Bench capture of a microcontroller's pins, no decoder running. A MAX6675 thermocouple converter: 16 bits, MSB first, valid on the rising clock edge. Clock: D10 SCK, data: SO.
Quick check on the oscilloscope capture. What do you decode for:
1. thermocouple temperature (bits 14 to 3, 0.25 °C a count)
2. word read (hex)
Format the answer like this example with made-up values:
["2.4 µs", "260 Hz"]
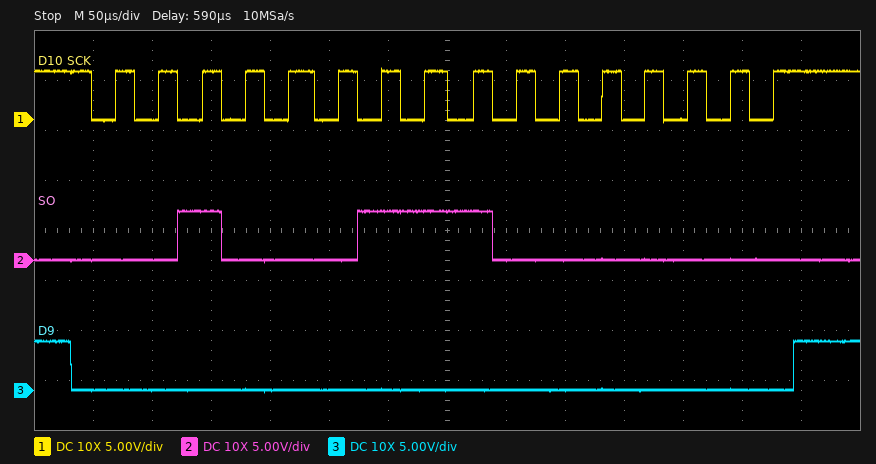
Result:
["284.00 °C", "0x2380"]
